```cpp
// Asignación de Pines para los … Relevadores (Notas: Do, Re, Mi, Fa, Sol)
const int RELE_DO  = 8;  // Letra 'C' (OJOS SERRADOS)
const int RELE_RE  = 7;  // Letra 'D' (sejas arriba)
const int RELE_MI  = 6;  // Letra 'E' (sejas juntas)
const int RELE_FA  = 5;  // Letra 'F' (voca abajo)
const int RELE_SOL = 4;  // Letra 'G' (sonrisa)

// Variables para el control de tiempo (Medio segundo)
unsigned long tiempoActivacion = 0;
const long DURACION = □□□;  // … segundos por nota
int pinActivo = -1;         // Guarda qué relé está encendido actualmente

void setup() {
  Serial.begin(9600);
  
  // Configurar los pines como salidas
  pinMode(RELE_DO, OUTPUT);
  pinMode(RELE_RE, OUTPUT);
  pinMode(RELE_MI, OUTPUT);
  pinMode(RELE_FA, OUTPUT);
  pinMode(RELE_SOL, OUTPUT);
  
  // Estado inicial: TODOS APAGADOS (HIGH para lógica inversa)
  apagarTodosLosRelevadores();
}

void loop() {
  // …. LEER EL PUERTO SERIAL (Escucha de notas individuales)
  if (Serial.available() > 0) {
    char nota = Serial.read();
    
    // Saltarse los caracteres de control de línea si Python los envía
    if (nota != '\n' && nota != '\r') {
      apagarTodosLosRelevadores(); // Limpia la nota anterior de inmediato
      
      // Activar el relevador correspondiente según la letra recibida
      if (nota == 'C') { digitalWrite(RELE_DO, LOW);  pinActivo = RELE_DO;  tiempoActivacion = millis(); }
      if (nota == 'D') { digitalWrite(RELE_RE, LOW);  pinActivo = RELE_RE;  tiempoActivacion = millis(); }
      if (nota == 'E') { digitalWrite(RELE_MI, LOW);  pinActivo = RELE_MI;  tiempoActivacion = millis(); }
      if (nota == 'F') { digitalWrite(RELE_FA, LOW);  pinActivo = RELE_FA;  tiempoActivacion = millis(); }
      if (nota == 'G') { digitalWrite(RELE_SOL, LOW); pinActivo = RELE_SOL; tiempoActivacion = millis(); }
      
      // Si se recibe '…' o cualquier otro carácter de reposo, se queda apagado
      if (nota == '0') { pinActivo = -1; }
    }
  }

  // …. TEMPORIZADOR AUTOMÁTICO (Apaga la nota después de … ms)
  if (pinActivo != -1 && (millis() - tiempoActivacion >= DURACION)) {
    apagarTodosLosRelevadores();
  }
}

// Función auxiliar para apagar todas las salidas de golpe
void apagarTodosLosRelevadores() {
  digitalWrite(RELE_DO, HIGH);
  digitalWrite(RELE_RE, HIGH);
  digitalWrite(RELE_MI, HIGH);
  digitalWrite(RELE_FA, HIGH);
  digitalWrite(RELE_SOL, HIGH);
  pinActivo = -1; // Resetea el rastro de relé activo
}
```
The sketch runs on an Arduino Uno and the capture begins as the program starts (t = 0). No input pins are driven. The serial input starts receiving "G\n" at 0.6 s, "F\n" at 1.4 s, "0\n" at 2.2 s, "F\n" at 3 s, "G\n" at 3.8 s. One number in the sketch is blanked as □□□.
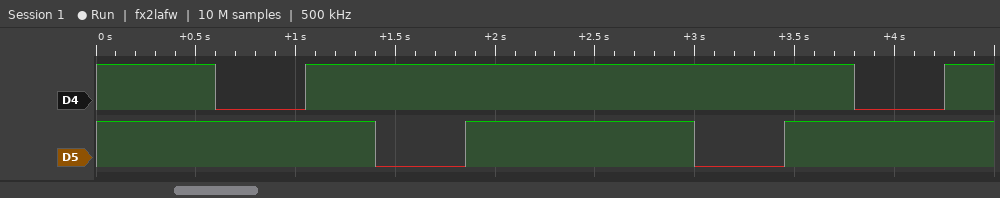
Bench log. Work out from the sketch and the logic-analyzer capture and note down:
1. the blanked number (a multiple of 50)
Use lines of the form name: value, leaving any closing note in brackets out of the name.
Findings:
the blanked number: 450
